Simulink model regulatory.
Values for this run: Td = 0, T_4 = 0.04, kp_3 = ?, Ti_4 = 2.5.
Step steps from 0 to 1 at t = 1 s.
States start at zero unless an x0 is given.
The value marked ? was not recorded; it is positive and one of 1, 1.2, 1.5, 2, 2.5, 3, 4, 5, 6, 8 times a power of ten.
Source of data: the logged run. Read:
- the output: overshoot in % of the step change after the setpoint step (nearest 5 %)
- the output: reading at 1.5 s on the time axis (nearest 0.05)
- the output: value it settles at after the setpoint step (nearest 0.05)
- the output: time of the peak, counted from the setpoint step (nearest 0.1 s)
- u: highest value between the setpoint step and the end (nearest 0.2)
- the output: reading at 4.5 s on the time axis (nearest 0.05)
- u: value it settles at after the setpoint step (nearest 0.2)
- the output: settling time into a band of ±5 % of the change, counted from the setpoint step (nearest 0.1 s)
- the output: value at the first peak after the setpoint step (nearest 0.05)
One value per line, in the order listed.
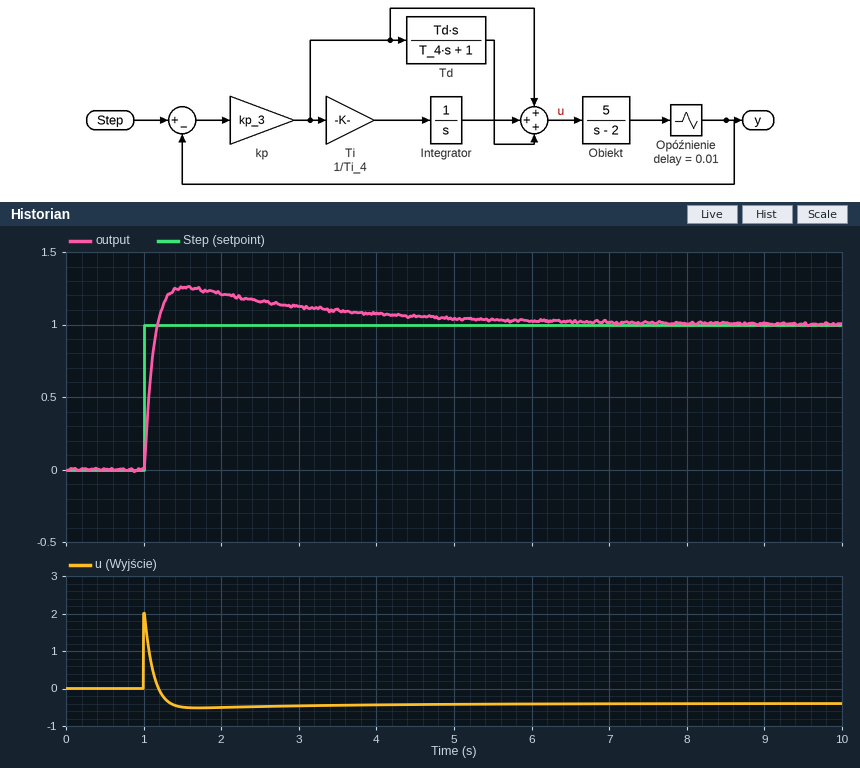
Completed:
25 %
1.25
1.00
0.5 s
2.0
1.05
-0.4
3.7 s
1.25
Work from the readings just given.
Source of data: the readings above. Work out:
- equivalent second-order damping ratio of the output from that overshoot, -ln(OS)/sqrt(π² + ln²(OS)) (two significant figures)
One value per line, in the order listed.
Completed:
0.40
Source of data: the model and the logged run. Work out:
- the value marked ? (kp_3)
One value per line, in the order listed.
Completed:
2
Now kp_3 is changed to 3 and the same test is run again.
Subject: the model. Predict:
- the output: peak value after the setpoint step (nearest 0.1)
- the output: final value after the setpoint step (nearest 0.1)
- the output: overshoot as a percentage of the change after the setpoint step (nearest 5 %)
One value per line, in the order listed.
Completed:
1.2
1.0
15 %
